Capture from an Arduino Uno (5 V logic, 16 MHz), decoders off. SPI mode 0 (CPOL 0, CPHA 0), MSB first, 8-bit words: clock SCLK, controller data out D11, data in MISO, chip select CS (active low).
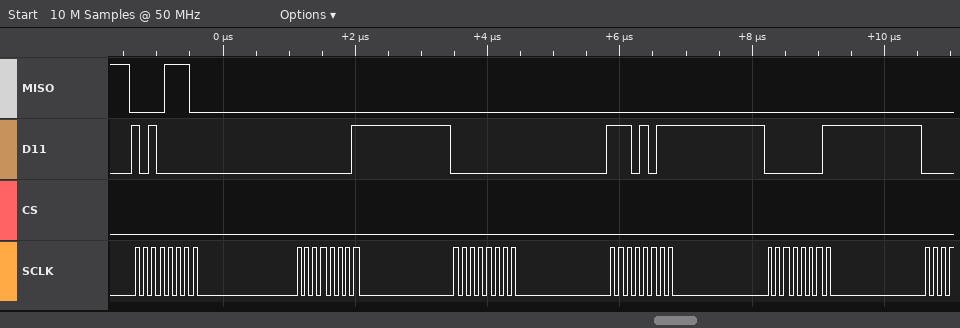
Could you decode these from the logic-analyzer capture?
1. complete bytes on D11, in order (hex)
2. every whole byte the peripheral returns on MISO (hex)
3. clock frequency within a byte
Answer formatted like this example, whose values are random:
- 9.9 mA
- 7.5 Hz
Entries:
- A0 01 00 EB 01
- 0E 00 00 00 00
- 8 MHz
